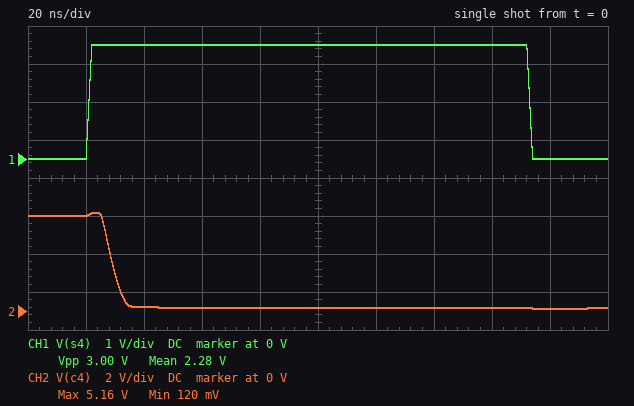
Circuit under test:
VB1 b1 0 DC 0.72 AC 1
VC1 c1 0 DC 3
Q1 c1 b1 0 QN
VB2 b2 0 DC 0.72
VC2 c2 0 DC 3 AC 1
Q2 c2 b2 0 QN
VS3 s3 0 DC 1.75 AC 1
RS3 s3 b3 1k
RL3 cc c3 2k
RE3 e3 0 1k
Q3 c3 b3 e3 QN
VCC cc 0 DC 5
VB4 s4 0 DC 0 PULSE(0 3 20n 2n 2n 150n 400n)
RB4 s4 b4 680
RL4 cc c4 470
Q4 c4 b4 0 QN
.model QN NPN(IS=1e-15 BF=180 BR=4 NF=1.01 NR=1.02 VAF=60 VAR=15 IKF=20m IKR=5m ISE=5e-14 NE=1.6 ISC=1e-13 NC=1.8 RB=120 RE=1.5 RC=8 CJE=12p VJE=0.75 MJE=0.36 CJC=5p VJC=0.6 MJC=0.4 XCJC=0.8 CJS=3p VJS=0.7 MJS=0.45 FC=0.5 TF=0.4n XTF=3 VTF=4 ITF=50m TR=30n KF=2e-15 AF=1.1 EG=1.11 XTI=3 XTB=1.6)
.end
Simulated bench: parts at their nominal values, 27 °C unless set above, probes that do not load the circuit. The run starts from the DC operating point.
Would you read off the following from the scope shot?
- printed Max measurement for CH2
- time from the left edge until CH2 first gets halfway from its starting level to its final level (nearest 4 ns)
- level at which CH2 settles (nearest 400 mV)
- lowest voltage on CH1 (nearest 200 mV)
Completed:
5.16 V
28 ns
0 V
0 V
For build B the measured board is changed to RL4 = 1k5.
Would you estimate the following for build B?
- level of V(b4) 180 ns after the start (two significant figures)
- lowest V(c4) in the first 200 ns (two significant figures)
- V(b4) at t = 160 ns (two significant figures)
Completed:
670 mV
36 mV
1.1 V
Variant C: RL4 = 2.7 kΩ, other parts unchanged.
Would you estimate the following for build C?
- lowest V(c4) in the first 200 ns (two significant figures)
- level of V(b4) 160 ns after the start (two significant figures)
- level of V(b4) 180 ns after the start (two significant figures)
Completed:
14 mV
1.1 V
660 mV
